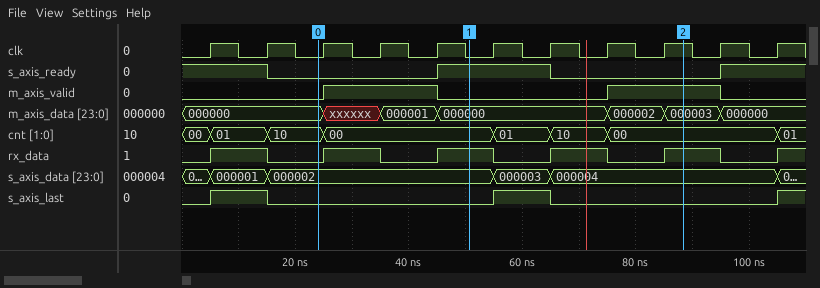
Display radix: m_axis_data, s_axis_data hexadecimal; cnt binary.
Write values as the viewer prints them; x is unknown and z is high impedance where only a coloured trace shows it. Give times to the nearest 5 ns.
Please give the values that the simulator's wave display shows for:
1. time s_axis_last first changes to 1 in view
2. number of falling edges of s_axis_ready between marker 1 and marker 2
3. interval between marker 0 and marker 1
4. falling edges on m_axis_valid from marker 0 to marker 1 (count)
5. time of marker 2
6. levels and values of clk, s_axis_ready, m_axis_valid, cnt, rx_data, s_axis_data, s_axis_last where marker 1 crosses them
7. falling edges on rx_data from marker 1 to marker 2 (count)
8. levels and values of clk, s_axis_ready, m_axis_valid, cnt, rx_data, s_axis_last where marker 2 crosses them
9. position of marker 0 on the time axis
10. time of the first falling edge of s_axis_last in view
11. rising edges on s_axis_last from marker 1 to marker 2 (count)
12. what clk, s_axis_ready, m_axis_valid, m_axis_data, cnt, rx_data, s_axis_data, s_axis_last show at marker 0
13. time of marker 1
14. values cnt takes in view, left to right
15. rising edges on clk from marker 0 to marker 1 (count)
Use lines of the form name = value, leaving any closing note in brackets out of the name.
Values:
time s_axis_last first changes to 1 in view = 5 ns
number of falling edges of s_axis_ready between marker 1 and marker 2 = 1
interval between marker 0 and marker 1 = 25 ns
falling edges on m_axis_valid from marker 0 to marker 1 = 1
time of marker 2 = 90 ns
levels and values of clk, s_axis_ready, m_axis_valid, cnt, rx_data, s_axis_data, s_axis_last where marker 1 crosses them = clk=0, s_axis_ready=1, m_axis_valid=0, cnt=00, rx_data=1, s_axis_data=000002, s_axis_last=0
falling edges on rx_data from marker 1 to marker 2 = 2
levels and values of clk, s_axis_ready, m_axis_valid, cnt, rx_data, s_axis_last where marker 2 crosses them = clk=1, s_axis_ready=0, m_axis_valid=1, cnt=00, rx_data=1, s_axis_last=0
position of marker 0 on the time axis = 25 ns
time of the first falling edge of s_axis_last in view = 15 ns
rising edges on s_axis_last from marker 1 to marker 2 = 1
what clk, s_axis_ready, m_axis_valid, m_axis_data, cnt, rx_data, s_axis_data, s_axis_last show at marker 0 = clk=0, s_axis_ready=0, m_axis_valid=0, m_axis_data=000000, cnt=10, rx_data=0, s_axis_data=000002, s_axis_last=0
time of marker 1 = 50 ns
values cnt takes in view, left to right = 00, 01, 10, 00, 01, 10, 00, 01
rising edges on clk from marker 0 to marker 1 = 3
